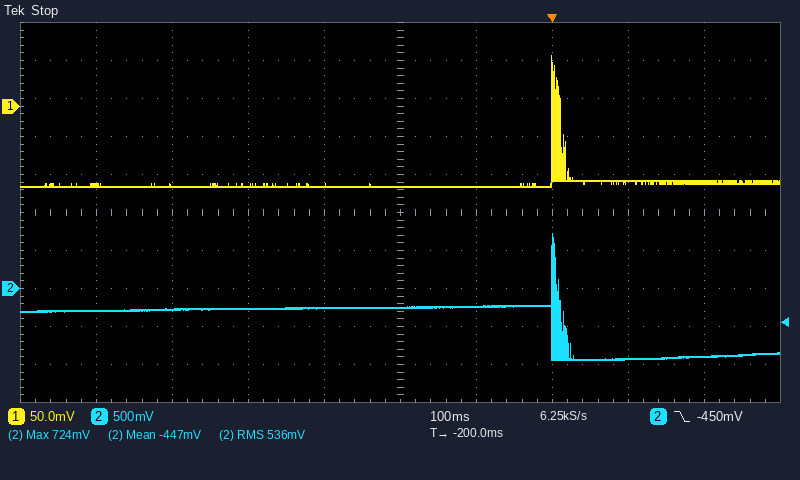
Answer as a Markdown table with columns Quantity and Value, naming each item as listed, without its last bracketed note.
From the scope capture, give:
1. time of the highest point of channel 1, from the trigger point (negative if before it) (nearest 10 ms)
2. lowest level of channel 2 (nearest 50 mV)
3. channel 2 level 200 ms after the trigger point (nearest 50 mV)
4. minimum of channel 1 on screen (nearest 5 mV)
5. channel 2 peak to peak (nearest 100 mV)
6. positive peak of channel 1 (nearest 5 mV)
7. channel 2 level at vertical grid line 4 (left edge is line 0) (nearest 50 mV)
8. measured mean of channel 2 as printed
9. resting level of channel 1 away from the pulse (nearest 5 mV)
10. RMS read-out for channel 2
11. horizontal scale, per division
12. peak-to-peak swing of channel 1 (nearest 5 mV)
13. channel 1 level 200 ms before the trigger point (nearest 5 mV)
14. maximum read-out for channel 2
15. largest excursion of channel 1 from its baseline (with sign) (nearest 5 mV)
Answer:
| Quantity | Value |
|---|---|
| time of the highest point of channel 1, from the trigger point (negative if before it) | 0 ms |
| lowest level of channel 2 | -950 mV |
| channel 2 level 200 ms after the trigger point | -900 mV |
| minimum of channel 1 on screen | -105 mV |
| channel 2 peak to peak | 1.70 V |
| positive peak of channel 1 | 65 mV |
| channel 2 level at vertical grid line 4 (left edge is line 0) | -250 mV |
| measured mean of channel 2 as printed | -447 mV |
| resting level of channel 1 away from the pulse | -105 mV |
| RMS read-out for channel 2 | 536 mV |
| horizontal scale, per division | 100 ms |
| peak-to-peak swing of channel 1 | 170 mV |
| channel 1 level 200 ms before the trigger point | -105 mV |
| maximum read-out for channel 2 | 724 mV |
| largest excursion of channel 1 from its baseline (with sign) | +170 mV |
